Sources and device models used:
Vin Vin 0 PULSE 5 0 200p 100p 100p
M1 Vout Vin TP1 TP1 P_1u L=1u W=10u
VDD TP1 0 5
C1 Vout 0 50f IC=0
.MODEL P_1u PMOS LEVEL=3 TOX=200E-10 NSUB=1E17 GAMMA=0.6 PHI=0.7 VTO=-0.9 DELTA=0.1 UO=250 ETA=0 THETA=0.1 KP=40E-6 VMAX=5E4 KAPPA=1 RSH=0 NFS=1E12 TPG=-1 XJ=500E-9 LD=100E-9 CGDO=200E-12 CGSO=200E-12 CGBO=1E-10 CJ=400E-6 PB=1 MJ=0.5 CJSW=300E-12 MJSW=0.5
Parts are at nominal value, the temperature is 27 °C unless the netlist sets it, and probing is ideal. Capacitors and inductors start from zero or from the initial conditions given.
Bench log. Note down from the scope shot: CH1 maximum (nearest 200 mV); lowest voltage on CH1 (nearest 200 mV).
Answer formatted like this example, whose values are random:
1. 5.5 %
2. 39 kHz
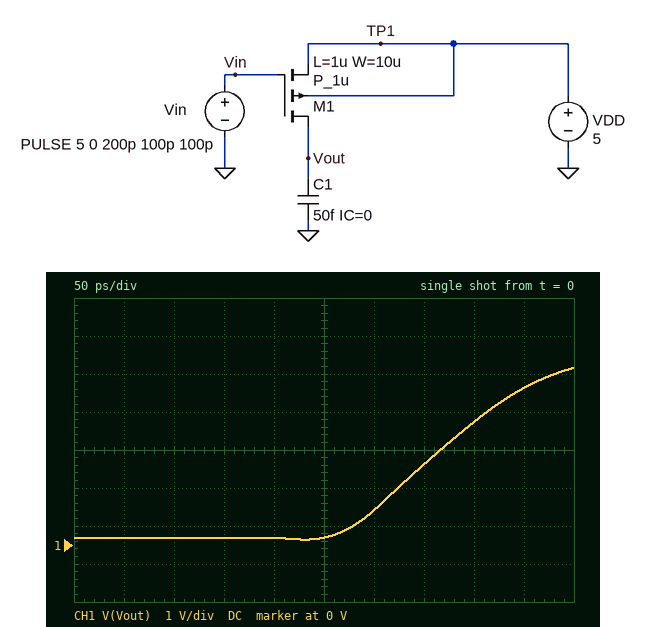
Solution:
1. 4.6 V
2. 200 mV
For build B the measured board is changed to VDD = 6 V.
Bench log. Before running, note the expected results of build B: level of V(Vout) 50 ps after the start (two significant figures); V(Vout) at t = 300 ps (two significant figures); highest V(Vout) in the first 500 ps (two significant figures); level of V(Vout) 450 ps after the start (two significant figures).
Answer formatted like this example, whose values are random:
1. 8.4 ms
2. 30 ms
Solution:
1. 200 mV
2. 1.6 V
3. 5.8 V
4. 5.4 V
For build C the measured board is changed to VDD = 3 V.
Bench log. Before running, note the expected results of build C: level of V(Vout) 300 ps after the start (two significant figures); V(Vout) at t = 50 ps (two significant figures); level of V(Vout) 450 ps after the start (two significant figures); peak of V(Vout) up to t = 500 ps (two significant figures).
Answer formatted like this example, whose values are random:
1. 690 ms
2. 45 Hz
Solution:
1. 170 mV
2. 190 mV
3. 1.6 V
4. 2.0 V
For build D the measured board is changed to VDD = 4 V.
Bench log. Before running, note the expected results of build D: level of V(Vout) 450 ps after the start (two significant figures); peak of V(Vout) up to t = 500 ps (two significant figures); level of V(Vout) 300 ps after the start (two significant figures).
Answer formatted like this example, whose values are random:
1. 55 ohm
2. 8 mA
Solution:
1. 2.8 V
2. 3.4 V
3. 460 mV
